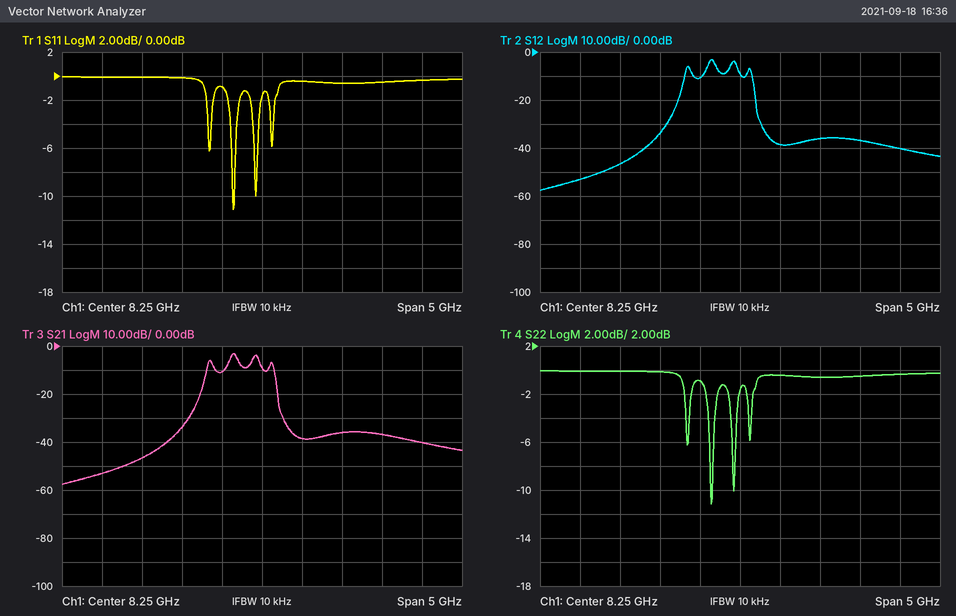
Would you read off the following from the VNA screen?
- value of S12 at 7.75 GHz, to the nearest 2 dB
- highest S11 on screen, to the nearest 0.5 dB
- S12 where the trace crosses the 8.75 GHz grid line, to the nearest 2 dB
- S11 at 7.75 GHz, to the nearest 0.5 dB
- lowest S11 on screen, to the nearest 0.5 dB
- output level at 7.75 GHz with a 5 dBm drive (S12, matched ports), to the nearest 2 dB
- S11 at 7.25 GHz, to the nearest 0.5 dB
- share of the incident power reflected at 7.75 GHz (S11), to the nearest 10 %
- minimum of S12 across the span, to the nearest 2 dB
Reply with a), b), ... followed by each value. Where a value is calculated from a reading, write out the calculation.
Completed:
a) -10 dB
b) 0.0 dB
c) -38 dB
d) -1.0 dB
e) -11.0 dB
f) 5 dBm + (-10 dB) = -6 dBm
g) 0.0 dB
h) 10^(-1/10) ≈ 79.4 %, so 80 % to the nearest 10 %
i) -58 dB
